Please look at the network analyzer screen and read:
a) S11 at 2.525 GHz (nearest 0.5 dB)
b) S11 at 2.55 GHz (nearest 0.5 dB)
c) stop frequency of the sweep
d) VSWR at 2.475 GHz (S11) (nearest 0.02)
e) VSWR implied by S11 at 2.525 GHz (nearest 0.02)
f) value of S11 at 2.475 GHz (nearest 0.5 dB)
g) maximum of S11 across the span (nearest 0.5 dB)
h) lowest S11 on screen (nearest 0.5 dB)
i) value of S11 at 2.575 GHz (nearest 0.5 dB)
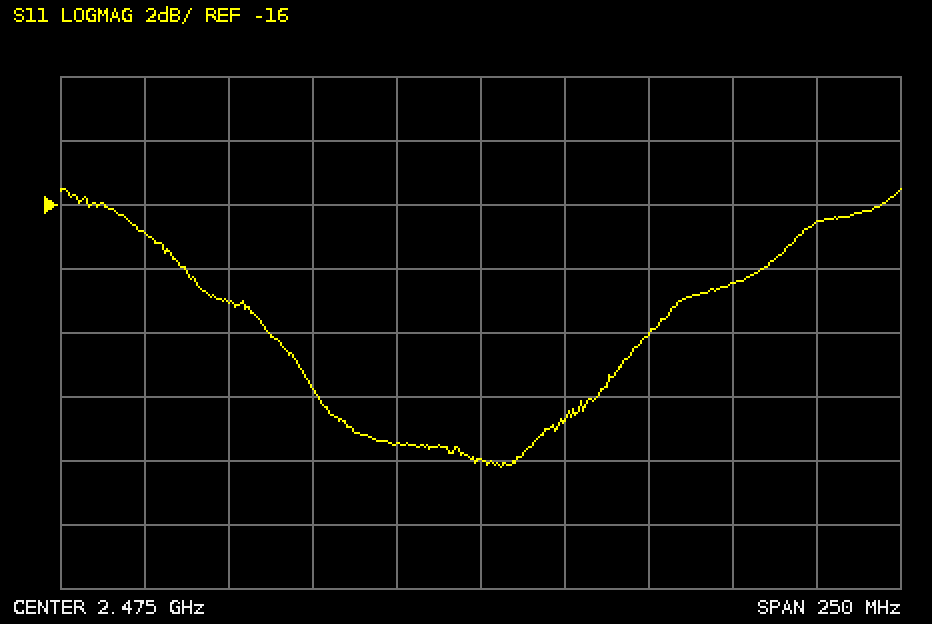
-20.0 dB
-18.5 dB
2.6 GHz
1.14
1.22
-24.0 dB
-15.5 dB
-24.0 dB
-16.5 dB
